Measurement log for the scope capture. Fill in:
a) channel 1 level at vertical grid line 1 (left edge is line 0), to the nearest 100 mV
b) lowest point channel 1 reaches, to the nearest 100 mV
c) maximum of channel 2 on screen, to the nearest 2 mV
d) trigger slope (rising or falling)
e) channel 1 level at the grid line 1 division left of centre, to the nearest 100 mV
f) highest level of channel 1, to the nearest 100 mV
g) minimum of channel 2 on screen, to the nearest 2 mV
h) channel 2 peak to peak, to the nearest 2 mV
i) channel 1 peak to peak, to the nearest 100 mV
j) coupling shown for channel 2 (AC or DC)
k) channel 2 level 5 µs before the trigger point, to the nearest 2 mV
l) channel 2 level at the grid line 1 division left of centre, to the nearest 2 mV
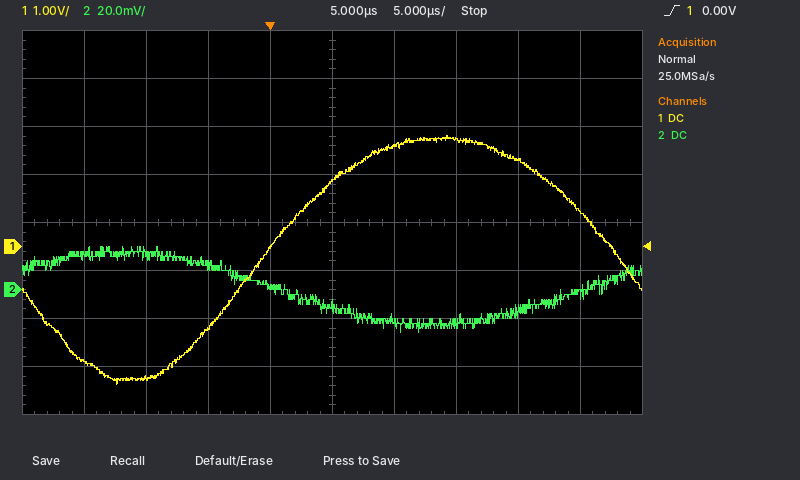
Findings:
-2.4 V
-2.9 V
18 mV
rising
0.0 V
2.3 V
-18 mV
36 mV
5.2 V
DC
10 mV
2 mV
